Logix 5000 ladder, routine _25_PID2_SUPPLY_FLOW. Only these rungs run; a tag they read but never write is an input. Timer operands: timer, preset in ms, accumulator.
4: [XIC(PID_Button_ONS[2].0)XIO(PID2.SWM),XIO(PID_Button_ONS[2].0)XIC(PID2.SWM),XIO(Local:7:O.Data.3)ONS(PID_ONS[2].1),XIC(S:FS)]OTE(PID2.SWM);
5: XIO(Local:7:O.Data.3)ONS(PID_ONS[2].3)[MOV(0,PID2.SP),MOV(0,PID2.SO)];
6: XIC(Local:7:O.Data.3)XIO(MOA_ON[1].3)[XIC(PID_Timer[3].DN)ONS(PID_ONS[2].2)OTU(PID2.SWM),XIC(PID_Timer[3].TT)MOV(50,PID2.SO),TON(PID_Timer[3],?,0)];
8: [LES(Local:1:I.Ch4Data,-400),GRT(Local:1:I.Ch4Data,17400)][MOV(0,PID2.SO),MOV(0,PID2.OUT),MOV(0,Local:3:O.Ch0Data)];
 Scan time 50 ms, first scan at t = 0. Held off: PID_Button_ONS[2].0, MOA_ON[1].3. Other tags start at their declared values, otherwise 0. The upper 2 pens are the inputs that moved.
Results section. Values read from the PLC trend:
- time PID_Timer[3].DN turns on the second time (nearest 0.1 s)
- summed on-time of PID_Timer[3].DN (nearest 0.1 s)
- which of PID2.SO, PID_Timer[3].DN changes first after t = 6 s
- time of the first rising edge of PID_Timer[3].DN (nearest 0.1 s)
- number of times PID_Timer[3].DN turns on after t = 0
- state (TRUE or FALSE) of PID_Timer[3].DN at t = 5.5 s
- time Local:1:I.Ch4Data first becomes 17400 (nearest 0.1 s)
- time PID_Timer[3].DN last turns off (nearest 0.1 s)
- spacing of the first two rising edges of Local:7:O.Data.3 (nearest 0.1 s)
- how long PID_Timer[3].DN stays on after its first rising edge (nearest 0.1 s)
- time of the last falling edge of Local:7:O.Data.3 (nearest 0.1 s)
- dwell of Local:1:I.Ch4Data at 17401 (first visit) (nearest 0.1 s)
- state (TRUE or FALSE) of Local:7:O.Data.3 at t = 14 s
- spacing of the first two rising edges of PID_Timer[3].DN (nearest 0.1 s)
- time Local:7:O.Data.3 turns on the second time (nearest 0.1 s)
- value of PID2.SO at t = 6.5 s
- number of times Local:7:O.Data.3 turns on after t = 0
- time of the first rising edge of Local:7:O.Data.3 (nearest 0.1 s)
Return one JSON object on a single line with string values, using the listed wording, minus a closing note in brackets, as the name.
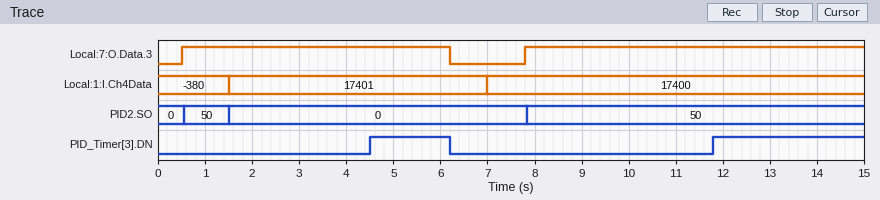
{"time PID_Timer[3].DN turns on the second time": "11.8 s", "summed on-time of PID_Timer[3].DN": "4.9 s", "which of PID2.SO, PID_Timer[3].DN changes first after t = 6 s": "PID_Timer[3].DN", "time of the first rising edge of PID_Timer[3].DN": "4.5 s", "number of times PID_Timer[3].DN turns on after t = 0": "2", "state (TRUE or FALSE) of PID_Timer[3].DN at t = 5.5 s": "TRUE", "time Local:1:I.Ch4Data first becomes 17400": "7.0 s", "time PID_Timer[3].DN last turns off": "6.2 s", "spacing of the first two rising edges of Local:7:O.Data.3": "7.3 s", "how long PID_Timer[3].DN stays on after its first rising edge": "1.7 s", "time of the last falling edge of Local:7:O.Data.3": "6.2 s", "dwell of Local:1:I.Ch4Data at 17401 (first visit)": "5.5 s", "state (TRUE or FALSE) of Local:7:O.Data.3 at t = 14 s": "TRUE", "spacing of the first two rising edges of PID_Timer[3].DN": "7.3 s", "time Local:7:O.Data.3 turns on the second time": "7.8 s", "value of PID2.SO at t = 6.5 s": "0", "number of times Local:7:O.Data.3 turns on after t = 0": "2", "time of the first rising edge of Local:7:O.Data.3": "0.5 s"}
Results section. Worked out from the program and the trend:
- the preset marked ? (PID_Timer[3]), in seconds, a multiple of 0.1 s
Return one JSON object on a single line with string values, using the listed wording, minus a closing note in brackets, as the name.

{"the preset marked ? (PID_Timer[3]), in seconds, a multiple of 0.1 s": "4.0 s"}
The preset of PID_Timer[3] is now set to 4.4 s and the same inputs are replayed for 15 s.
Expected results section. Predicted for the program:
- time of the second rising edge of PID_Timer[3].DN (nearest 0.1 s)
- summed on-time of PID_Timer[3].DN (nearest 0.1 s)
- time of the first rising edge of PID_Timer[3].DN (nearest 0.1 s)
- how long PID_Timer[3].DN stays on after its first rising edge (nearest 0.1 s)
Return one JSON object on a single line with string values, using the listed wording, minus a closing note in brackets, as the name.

{"time of the second rising edge of PID_Timer[3].DN": "12.2 s", "summed on-time of PID_Timer[3].DN": "4.1 s", "time of the first rising edge of PID_Timer[3].DN": "4.9 s", "how long PID_Timer[3].DN stays on after its first rising edge": "1.3 s"}
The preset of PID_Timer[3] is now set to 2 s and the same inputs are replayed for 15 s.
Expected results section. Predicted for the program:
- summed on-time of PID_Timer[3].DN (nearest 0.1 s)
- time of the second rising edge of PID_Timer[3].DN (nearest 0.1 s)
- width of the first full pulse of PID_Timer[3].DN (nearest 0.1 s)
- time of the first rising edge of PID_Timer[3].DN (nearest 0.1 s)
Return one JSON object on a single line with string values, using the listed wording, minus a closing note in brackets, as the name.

{"summed on-time of PID_Timer[3].DN": "8.9 s", "time of the second rising edge of PID_Timer[3].DN": "9.8 s", "width of the first full pulse of PID_Timer[3].DN": "3.7 s", "time of the first rising edge of PID_Timer[3].DN": "2.5 s"}
